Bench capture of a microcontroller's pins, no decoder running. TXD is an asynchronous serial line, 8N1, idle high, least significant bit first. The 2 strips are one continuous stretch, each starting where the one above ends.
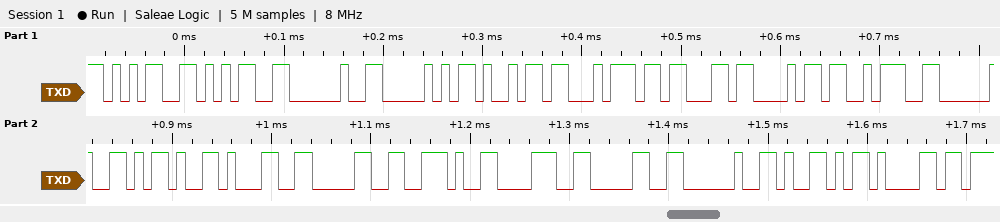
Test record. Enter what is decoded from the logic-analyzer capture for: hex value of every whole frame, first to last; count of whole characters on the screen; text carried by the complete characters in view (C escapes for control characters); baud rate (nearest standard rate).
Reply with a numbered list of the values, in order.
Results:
1. 0x35 0x35 0x20 0x50 0x69 0x74 0x63 0x68 0x3A 0x20 0x2D 0x31 0x30 0x2E 0x38 0x30 0x20 0x59 0x61
2. 19
3. "55 Pitch: -10.80 Ya"
4. 115200 baud
